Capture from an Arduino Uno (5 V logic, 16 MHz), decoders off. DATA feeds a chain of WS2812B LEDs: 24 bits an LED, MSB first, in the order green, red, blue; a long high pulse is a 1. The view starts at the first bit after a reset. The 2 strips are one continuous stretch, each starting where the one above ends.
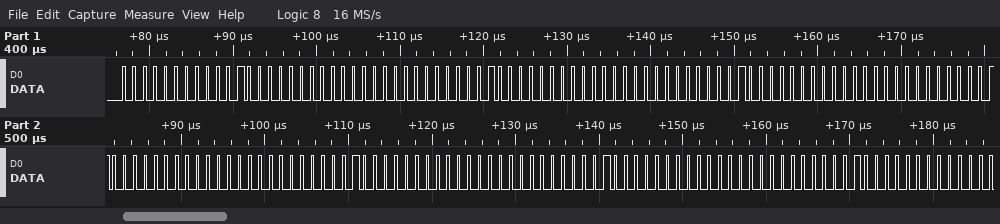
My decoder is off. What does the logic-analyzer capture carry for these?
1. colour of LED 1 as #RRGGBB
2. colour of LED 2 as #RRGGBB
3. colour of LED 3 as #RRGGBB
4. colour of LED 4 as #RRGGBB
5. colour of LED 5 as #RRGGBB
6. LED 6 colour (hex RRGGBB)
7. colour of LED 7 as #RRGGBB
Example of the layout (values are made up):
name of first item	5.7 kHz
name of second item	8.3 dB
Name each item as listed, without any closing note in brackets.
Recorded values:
colour of LED 1 as #RRGGBB	#100000
colour of LED 2 as #RRGGBB	#100000
colour of LED 3 as #RRGGBB	#100000
colour of LED 4 as #RRGGBB	#100000
colour of LED 5 as #RRGGBB	#100000
LED 6 colour	#100000
colour of LED 7 as #RRGGBB	#100000
